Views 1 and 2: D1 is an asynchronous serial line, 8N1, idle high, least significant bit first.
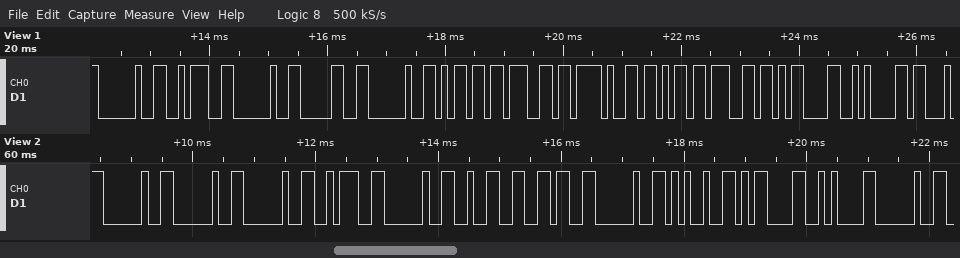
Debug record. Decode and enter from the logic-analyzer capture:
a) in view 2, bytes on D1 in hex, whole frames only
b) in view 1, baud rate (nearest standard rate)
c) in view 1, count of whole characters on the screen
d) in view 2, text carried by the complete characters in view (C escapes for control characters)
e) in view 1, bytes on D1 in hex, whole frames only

20 20 20 3A 20 32 36 20 25 0D 0A 20
9600 baud
12
"   : 26 %\r\n "
20 3A 20 30 20 6D 67 2F 6B 67 0D 0A
